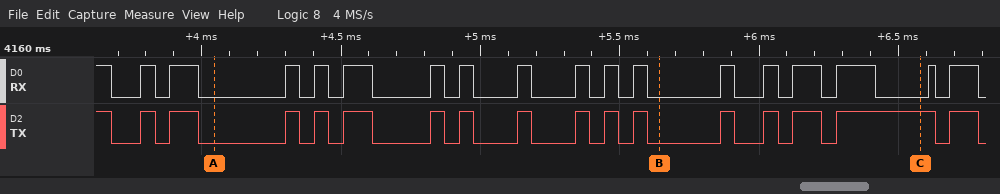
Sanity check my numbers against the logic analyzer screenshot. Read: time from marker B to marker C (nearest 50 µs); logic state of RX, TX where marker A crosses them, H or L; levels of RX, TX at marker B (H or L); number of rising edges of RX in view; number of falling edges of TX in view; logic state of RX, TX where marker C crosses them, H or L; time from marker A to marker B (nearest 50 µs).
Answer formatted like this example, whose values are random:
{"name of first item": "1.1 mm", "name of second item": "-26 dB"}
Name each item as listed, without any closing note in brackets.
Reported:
{"time from marker B to marker C": "950 µs", "logic state of RX, TX where marker A crosses them, H or L": "RX=L, TX=L", "levels of RX, TX at marker B": "RX=L, TX=L", "number of rising edges of RX in view": "17", "number of falling edges of TX in view": "17", "logic state of RX, TX where marker C crosses them, H or L": "RX=L, TX=H", "time from marker A to marker B": "1600 µs"}
